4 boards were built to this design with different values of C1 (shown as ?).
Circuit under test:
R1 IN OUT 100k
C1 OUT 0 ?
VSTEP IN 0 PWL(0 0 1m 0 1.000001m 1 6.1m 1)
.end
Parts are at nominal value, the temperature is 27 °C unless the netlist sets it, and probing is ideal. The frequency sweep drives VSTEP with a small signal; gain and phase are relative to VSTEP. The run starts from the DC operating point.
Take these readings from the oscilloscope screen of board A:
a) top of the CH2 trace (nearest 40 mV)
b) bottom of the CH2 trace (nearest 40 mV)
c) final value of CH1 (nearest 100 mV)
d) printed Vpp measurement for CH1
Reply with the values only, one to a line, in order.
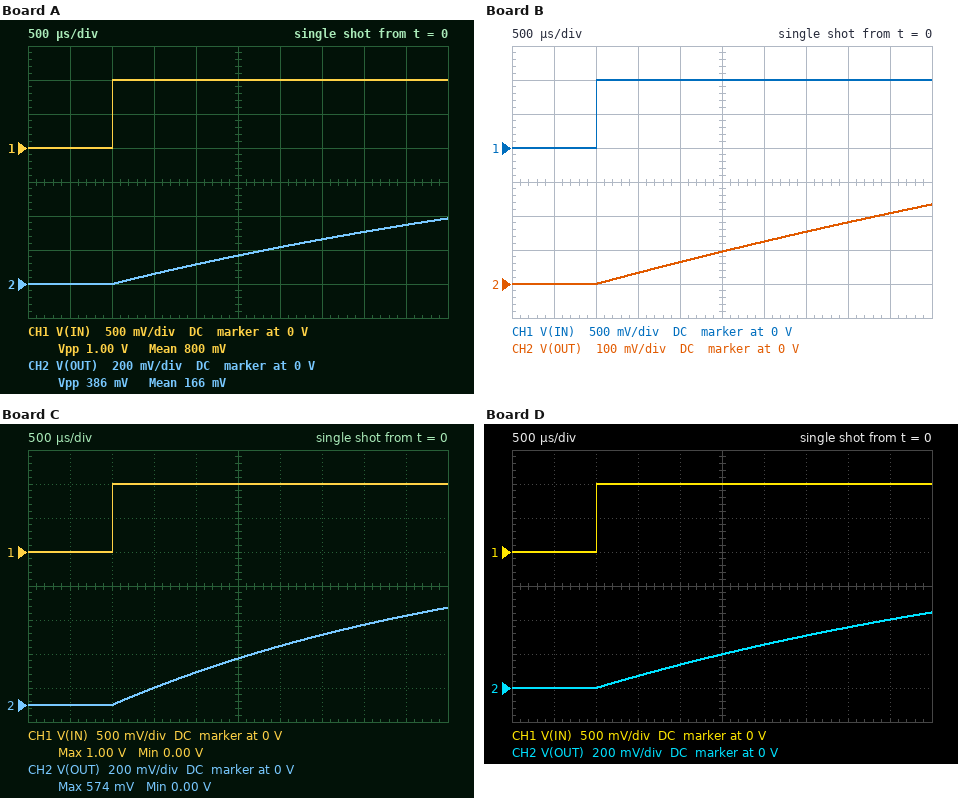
400 mV
0 V
1.0 V
1.00 V
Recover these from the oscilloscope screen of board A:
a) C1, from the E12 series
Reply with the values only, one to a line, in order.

82 nF
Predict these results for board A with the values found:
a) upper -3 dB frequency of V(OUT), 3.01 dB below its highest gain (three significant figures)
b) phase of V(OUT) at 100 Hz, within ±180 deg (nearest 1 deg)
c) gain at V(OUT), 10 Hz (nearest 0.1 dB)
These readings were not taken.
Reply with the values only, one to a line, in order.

19.4 Hz
-79 deg
-1.0 dB
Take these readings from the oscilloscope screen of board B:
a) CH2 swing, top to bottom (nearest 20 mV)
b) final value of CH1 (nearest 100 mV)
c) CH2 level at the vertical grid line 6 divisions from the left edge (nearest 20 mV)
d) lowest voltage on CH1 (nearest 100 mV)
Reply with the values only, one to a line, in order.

240 mV
1.0 V
120 mV
0 V
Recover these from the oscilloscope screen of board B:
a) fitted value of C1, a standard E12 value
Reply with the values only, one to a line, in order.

150 nF
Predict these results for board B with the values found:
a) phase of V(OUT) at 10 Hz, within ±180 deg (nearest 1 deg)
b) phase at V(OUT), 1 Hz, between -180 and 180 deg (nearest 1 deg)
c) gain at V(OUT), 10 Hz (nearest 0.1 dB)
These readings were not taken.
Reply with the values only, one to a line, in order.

-43 deg
-5 deg
-2.8 dB
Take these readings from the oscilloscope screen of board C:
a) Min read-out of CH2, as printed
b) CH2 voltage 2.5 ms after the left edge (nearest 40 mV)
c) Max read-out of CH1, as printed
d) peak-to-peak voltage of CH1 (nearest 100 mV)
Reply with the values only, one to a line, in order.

0.00 V
280 mV
1.00 V
1.0 V
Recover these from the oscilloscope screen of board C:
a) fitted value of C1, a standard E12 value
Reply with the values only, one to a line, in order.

47 nF
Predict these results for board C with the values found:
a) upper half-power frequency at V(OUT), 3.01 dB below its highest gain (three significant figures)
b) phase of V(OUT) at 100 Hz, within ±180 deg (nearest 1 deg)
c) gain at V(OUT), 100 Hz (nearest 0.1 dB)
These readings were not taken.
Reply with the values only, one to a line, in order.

33.9 Hz
-71 deg
-9.9 dB
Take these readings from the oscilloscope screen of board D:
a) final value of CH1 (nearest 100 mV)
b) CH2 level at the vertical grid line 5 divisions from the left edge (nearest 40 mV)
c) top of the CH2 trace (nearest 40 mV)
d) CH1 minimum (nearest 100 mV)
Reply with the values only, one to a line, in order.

1.0 V
200 mV
440 mV
0 V
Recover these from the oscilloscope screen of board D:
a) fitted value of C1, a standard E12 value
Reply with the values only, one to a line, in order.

68 nF
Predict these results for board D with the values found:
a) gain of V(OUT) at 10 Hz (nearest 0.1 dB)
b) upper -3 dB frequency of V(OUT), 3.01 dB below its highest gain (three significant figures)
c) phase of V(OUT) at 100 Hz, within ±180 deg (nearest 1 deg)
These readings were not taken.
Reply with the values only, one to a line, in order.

-0.7 dB
23.4 Hz
-77 deg
